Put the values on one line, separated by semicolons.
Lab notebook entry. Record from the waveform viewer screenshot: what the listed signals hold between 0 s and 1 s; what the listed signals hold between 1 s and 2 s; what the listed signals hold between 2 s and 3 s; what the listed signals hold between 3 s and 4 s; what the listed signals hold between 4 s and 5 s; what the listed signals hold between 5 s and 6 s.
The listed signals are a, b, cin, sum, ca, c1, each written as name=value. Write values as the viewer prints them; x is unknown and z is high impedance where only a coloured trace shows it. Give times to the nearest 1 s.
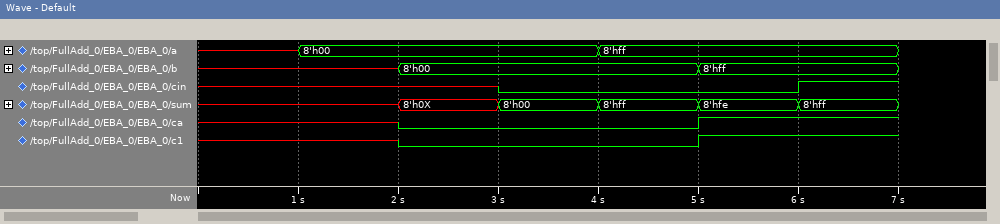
a=x, b=x, cin=x, sum=x, ca=x, c1=x; a=8'h00, b=x, cin=x, sum=x, ca=x, c1=x; a=8'h00, b=8'h00, cin=x, sum=8'h0X, ca=0, c1=0; a=8'h00, b=8'h00, cin=0, sum=8'h00, ca=0, c1=0; a=8'hff, b=8'h00, cin=0, sum=8'hff, ca=0, c1=0; a=8'hff, b=8'hff, cin=0, sum=8'hfe, ca=1, c1=1
